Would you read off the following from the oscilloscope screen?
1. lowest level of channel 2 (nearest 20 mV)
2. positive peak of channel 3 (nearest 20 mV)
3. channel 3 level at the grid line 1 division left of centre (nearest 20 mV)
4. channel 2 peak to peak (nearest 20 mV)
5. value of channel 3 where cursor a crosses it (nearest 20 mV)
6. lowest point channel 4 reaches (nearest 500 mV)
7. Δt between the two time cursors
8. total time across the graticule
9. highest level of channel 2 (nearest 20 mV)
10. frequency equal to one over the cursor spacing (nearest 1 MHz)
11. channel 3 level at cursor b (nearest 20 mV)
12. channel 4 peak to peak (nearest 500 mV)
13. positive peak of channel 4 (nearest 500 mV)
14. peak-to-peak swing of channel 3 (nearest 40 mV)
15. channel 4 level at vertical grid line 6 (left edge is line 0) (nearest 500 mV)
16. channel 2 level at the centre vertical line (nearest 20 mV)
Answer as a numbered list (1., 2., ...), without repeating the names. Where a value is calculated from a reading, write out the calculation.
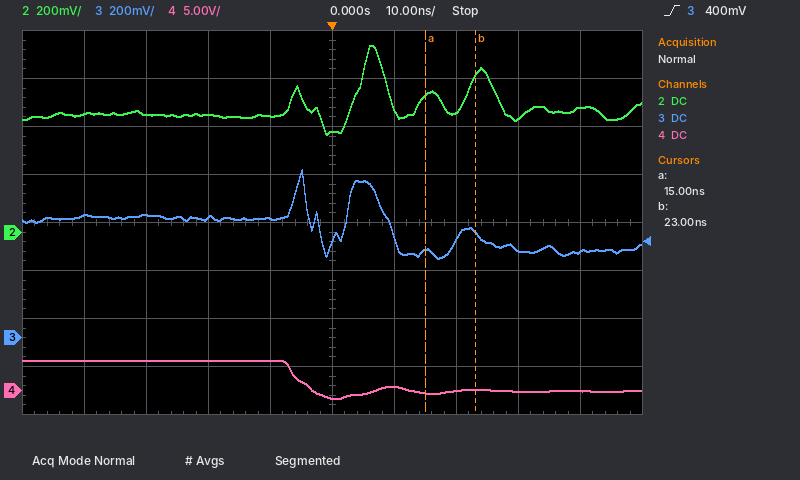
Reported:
1. 400 mV
2. 700 mV
3. 500 mV
4. 780 mV − (400 mV) = 380 mV
5. 360 mV
6. -1.0 V
7. 23 ns − (15 ns) = 8 ns
8. 100 ns
9. 780 mV
10. 1 / 8 ns ≈ 125 MHz
11. 440 mV
12. 3.0 V − (-1.0 V) = 4.0 V
13. 3.0 V
14. 360 mV
15. 500 mV
16. 420 mV
